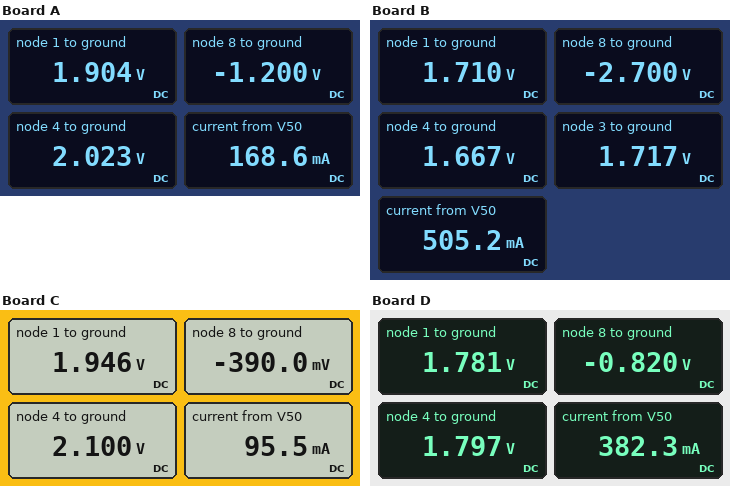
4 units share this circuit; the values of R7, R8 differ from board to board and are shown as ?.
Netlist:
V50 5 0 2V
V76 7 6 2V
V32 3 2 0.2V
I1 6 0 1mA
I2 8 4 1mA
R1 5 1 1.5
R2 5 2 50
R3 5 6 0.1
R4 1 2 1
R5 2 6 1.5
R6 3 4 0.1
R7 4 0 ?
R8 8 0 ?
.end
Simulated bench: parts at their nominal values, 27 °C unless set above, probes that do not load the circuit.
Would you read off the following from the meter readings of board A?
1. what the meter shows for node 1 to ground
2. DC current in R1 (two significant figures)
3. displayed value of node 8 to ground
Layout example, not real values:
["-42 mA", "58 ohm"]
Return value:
["1.904 V", "64 mA", "-1.200 V"]
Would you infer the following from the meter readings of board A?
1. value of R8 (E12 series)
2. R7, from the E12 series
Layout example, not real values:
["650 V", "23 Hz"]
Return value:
["1.2 kΩ", "12 Ω"]
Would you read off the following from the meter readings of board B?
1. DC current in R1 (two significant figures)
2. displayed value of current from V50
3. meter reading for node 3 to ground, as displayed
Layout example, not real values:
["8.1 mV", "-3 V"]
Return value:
["190 mA", "505.2 mA", "1.717 V"]
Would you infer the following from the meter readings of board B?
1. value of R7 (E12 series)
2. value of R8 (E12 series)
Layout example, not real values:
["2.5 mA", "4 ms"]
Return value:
["3.3 Ω", "2.7 kΩ"]
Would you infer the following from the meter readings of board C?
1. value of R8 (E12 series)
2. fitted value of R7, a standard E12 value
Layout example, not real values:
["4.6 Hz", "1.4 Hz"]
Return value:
["390 Ω", "22 Ω"]
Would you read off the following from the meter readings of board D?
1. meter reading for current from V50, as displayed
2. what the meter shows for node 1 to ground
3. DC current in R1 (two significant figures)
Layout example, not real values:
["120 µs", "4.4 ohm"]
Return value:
["382.3 mA", "1.781 V", "150 mA"]
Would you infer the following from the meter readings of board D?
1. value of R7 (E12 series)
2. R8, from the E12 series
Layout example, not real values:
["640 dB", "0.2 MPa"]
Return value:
["4.7 Ω", "820 Ω"]
